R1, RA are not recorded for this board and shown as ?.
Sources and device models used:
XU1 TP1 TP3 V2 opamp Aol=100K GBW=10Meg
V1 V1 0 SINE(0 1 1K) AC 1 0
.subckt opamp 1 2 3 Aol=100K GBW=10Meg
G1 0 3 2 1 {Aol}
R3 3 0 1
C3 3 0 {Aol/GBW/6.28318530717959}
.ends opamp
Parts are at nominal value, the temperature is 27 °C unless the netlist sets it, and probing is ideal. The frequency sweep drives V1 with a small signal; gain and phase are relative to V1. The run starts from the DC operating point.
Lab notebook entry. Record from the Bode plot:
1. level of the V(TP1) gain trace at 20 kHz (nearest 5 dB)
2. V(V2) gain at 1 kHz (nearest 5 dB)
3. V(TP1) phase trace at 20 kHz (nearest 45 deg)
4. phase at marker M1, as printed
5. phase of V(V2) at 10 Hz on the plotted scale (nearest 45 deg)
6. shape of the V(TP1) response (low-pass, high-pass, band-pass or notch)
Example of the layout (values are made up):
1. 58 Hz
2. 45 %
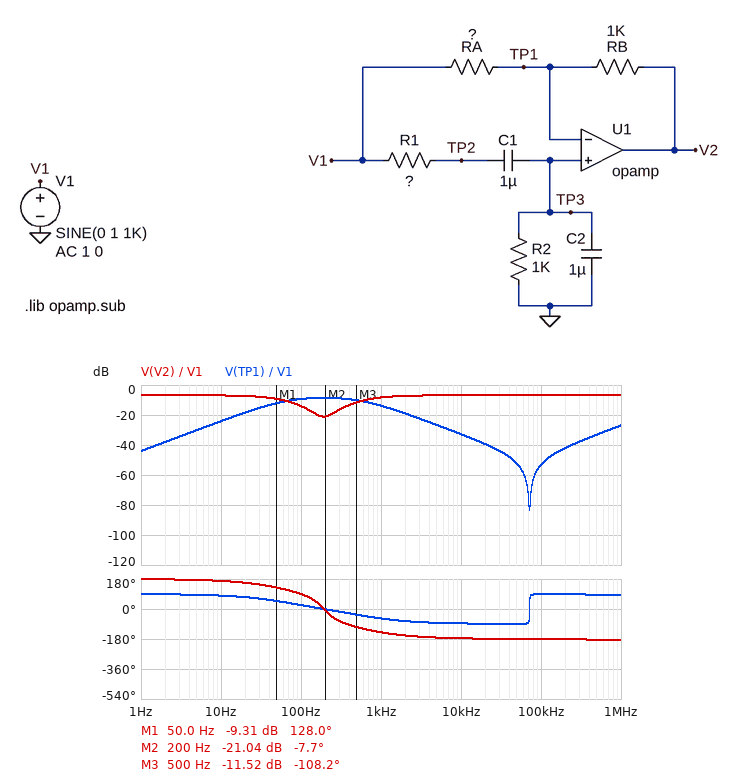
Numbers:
1. -40 dB
2. -10 dB
3. -90 deg
4. 128.0 deg
5. 180 deg
6. band-pass
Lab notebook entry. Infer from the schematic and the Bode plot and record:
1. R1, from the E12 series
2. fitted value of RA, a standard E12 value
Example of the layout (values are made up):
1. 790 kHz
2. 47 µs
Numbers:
1. 680 Ω
2. 2.2 kΩ
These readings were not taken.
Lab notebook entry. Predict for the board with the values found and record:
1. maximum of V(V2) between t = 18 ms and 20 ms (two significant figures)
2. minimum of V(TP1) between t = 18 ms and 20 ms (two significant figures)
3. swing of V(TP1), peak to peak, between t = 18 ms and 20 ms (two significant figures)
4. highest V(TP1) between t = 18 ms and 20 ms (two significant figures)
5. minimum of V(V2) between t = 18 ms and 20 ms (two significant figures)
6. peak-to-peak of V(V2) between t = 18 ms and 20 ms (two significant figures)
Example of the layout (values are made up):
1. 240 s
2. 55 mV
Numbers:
1. 380 mV
2. -200 mV
3. 410 mV
4. 200 mV
5. -380 mV
6. 770 mV
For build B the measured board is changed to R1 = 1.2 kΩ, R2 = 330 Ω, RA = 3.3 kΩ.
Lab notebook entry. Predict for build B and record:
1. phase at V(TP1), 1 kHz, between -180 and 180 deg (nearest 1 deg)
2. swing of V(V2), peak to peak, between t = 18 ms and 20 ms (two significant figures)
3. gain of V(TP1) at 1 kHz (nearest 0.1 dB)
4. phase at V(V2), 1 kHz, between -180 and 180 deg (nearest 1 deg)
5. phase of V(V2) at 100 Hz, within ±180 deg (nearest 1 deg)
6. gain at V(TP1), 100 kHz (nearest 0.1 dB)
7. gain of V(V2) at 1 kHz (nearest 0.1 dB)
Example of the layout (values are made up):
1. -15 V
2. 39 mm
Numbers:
1. -51 deg
2. 480 mV
3. -19.1 dB
4. -152 deg
5. 144 deg
6. -55.4 dB
7. -12.4 dB
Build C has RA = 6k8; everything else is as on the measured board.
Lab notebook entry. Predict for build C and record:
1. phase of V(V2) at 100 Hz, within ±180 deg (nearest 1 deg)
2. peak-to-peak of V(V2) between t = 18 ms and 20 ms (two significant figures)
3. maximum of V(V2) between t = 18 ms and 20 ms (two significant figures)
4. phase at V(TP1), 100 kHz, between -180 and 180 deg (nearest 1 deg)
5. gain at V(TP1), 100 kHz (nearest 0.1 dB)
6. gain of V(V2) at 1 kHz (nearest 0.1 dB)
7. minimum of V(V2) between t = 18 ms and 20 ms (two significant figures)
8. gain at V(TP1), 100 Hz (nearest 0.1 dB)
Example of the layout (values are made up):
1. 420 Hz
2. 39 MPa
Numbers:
1. 36 deg
2. 390 mV
3. 200 mV
4. -90 deg
5. -61.2 dB
6. -14.1 dB
7. -200 mV
8. -9.3 dB
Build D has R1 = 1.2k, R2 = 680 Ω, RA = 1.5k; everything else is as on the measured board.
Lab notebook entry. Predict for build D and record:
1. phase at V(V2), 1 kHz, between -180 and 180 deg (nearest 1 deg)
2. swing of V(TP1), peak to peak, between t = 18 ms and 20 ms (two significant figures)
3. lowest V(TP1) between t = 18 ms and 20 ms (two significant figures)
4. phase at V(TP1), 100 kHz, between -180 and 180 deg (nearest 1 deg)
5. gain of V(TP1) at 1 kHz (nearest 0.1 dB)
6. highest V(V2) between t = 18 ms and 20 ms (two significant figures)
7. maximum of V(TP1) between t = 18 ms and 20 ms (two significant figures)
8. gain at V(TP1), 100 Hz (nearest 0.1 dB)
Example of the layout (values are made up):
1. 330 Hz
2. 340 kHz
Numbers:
1. -163 deg
2. 240 mV
3. -120 mV
4. 89 deg
5. -18.3 dB
6. 600 mV
7. 120 mV
8. -12.2 dB
